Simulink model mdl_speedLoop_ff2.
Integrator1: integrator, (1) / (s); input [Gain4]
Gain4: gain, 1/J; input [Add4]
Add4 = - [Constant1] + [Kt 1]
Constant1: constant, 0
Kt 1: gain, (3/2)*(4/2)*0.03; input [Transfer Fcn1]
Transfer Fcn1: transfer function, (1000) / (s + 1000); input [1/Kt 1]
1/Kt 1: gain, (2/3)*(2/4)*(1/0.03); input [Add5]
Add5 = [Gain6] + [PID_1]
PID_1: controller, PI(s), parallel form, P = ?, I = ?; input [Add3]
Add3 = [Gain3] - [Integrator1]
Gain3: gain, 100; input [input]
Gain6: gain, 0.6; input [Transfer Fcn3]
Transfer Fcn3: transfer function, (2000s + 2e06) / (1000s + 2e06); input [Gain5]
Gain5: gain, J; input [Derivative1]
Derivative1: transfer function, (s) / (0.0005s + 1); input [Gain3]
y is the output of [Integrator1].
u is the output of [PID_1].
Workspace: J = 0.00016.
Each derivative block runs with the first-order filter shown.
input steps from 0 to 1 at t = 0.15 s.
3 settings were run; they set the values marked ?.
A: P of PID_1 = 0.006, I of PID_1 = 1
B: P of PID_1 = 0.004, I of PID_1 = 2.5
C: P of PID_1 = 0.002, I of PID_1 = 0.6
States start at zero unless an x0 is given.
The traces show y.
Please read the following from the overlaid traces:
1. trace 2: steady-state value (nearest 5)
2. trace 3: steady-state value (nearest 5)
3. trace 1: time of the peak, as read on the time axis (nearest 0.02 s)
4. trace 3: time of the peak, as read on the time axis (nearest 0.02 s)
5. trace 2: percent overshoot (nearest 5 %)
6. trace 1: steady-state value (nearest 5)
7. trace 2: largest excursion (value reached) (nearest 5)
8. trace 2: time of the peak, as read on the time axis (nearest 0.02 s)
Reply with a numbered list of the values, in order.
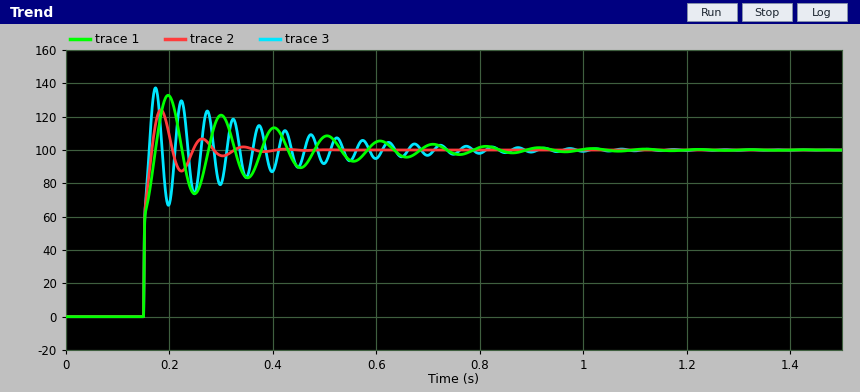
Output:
1. 100
2. 100
3. 0.20 s
4. 0.18 s
5. 25 %
6. 100
7. 125
8. 0.18 s
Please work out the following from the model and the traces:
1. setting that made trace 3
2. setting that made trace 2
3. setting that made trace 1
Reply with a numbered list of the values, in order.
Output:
1. B
2. A
3. C
